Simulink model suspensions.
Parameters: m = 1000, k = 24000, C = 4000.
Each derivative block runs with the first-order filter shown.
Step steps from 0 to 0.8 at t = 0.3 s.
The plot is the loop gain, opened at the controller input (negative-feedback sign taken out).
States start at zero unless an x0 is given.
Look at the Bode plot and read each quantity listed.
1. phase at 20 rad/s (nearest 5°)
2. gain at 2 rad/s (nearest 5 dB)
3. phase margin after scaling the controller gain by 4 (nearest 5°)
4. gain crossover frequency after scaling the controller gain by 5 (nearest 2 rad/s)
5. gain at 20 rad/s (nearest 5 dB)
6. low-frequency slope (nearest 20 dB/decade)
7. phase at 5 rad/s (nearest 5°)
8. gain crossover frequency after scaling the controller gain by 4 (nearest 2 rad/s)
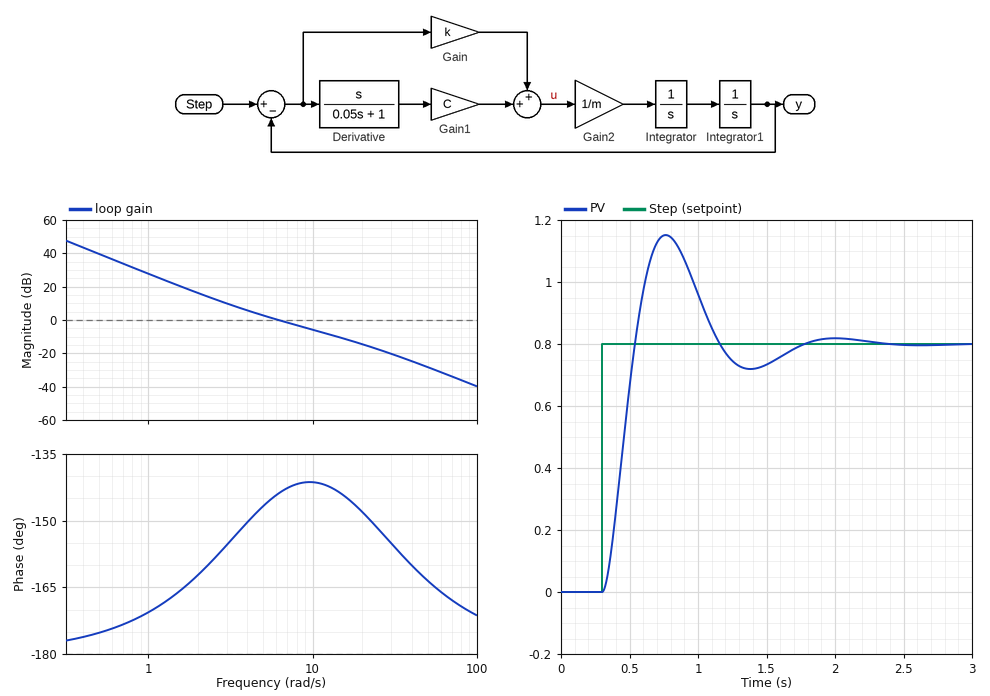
-150°
15 dB
35°
20 rad/s
-15 dB
-40 dB/decade
-145°
16 rad/s
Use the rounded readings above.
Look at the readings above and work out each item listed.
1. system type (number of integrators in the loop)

2
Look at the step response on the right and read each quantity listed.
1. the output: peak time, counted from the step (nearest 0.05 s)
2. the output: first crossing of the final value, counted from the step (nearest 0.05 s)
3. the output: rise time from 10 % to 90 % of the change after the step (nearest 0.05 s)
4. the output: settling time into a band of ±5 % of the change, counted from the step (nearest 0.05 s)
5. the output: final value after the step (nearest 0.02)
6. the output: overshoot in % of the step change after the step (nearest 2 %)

0.45 s
0.25 s
0.15 s
1.30 s
0.80
44 %
